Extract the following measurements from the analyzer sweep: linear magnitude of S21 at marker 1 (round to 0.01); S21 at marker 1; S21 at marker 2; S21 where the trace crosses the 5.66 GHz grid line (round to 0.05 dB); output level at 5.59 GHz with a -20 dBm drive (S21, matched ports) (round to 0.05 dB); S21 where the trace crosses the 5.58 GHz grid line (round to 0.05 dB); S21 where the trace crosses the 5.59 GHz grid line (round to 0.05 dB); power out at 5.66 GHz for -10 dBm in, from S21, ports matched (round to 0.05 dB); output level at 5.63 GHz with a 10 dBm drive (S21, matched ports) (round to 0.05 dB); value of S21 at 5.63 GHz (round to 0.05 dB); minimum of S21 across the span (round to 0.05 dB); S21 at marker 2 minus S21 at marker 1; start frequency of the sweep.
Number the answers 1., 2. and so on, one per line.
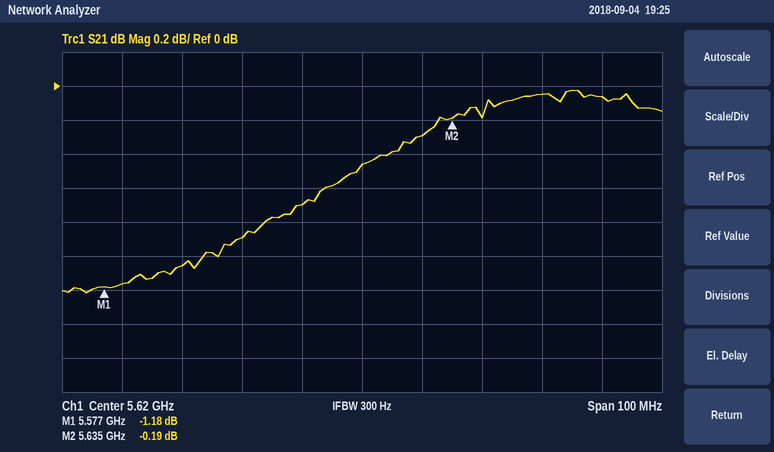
1. 0.87
2. -1.18 dB
3. -0.19 dB
4. -0.05 dB
5. -21.05 dBm
6. -1.15 dB
7. -1.05 dB
8. -10.05 dBm
9. 9.70 dBm
10. -0.30 dB
11. -1.20 dB
12. 0.99 dB
13. 5.57 GHz
